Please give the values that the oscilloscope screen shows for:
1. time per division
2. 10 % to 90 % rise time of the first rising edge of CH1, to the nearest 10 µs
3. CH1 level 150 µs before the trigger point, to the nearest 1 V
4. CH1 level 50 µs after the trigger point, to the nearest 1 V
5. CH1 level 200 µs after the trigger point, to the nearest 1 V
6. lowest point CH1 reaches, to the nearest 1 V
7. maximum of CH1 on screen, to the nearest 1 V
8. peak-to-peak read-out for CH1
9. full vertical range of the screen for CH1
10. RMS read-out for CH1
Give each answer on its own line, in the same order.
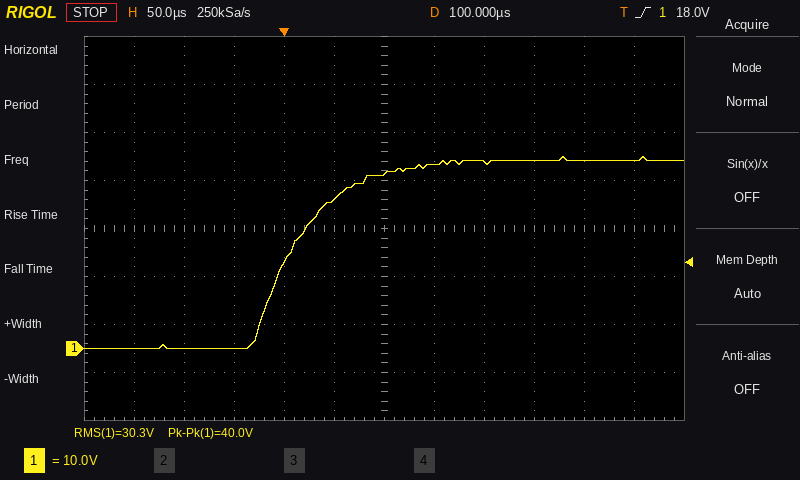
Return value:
50 µs
110 µs
0 V
31 V
39 V
0 V
40 V
40.0 V
80 V
30.3 V
